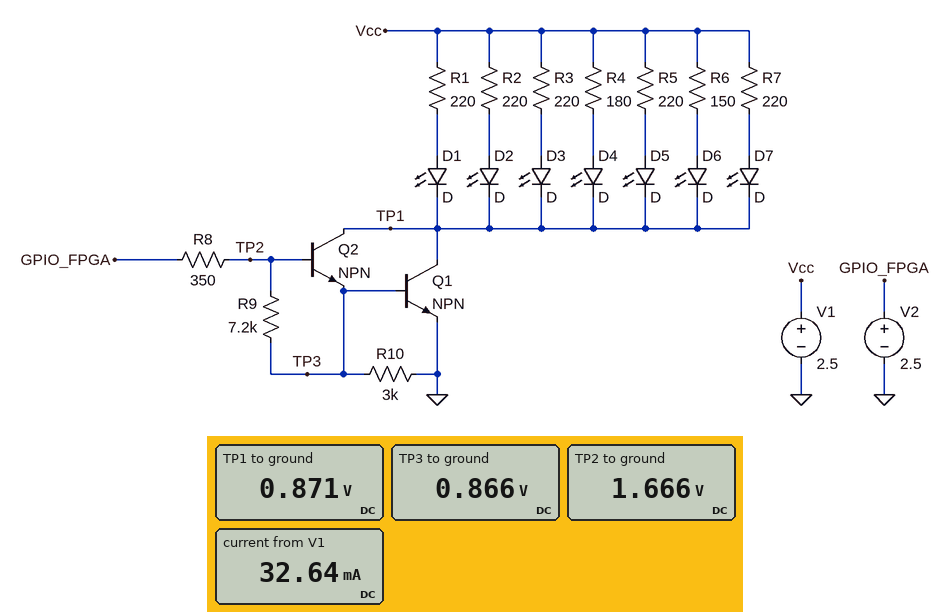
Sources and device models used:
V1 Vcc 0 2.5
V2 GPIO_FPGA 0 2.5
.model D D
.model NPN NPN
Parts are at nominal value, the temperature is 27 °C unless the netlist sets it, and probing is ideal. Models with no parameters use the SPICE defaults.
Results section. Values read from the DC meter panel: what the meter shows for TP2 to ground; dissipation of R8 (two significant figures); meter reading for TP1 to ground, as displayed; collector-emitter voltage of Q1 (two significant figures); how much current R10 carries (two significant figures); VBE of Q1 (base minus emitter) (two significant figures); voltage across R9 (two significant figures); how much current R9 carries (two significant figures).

1.666 V
2.0 mW
0.871 V
870 mV
290 µA
870 mV
800 mV
110 µA
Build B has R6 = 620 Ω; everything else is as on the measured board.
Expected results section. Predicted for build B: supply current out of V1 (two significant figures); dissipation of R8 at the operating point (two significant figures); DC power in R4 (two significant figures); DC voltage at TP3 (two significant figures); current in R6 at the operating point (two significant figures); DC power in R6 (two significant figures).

28 mA
2.0 mW
4.9 mW
860 mV
1.6 mA
1.5 mW
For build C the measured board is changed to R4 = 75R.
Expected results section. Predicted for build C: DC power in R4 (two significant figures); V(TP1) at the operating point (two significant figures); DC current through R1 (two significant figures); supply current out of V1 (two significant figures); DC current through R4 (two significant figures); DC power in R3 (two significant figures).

11 mW
880 mV
4.2 mA
39 mA
12 mA
3.9 mW
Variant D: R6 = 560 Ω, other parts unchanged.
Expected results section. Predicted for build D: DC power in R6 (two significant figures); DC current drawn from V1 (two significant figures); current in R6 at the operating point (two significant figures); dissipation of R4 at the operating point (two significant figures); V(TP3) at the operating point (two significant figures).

1.7 mW
28 mA
1.7 mA
4.9 mW
860 mV
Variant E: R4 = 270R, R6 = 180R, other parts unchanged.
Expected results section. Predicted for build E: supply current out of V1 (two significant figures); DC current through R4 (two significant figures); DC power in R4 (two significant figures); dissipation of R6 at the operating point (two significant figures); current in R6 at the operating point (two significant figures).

30 mA
3.5 mA
3.3 mW
4.8 mW
5.2 mA
